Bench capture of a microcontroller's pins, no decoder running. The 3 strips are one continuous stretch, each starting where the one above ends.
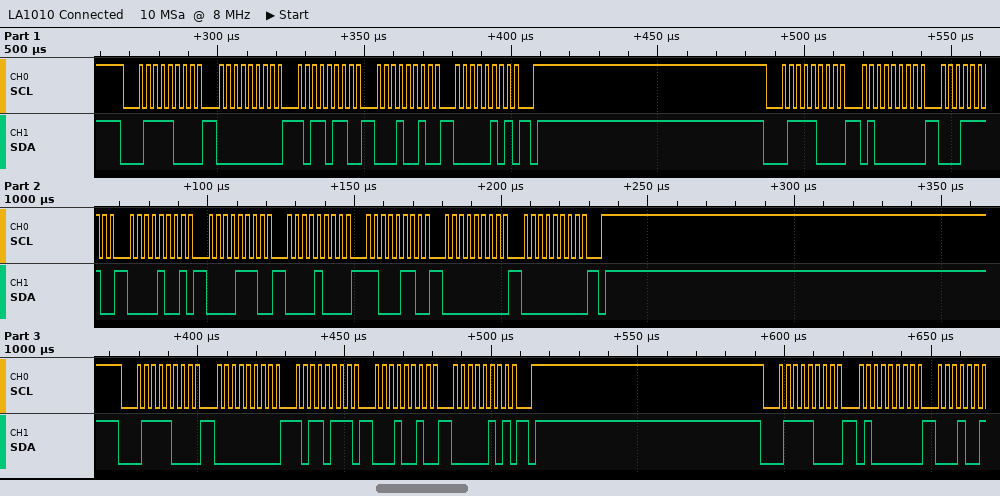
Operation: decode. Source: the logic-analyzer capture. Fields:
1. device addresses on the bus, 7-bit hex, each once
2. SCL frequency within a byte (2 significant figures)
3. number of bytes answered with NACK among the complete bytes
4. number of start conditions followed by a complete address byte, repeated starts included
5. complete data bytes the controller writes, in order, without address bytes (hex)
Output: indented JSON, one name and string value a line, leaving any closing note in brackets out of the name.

{
  "device addresses on the bus, 7-bit hex, each once": "0x3C",
  "SCL frequency within a byte": "400 kHz",
  "number of bytes answered with NACK among the complete bytes": "0",
  "number of start conditions followed by a complete address byte, repeated starts included": "4",
  "complete data bytes the controller writes, in order, without address bytes": "00 B6 12 05 40 1E 09 0E 08 C6 00 00 00 B7 12 05 40"
}
